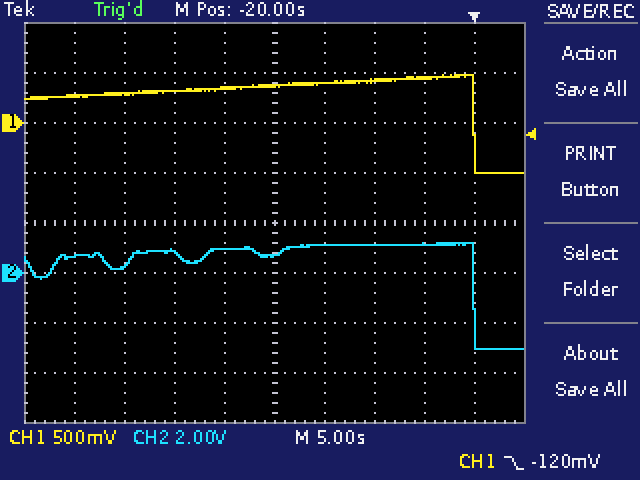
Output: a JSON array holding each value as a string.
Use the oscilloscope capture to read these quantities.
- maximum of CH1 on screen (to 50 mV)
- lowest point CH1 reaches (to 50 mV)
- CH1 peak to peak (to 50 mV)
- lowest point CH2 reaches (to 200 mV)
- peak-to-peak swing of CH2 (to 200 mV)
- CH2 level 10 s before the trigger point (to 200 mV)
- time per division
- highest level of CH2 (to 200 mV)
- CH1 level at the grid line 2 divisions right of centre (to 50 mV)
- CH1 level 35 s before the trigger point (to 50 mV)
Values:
["500 mV", "-500 mV", "1.00 V", "-3.0 V", "4.2 V", "1.2 V", "5 s", "1.2 V", "400 mV", "300 mV"]
